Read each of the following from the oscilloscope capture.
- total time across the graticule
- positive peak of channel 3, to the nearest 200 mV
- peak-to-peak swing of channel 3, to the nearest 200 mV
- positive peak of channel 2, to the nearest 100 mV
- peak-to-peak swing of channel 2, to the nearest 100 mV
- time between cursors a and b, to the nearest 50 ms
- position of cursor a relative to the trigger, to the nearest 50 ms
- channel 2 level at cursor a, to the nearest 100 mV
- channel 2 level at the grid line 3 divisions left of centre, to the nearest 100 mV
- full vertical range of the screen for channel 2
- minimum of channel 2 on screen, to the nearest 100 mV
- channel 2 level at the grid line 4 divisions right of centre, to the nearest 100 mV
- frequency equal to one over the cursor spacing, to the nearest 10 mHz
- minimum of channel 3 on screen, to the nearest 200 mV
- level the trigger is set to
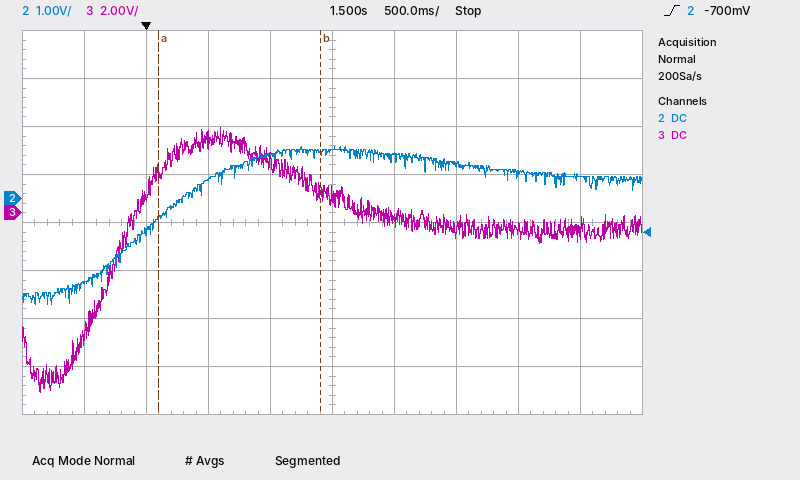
5 s
3.6 V
11.0 V
1.1 V
3.3 V
1.30 s
+100 ms
-400 mV
-700 mV
8 V
-2.2 V
500 mV
770 mHz
-7.4 V
-700 mV
